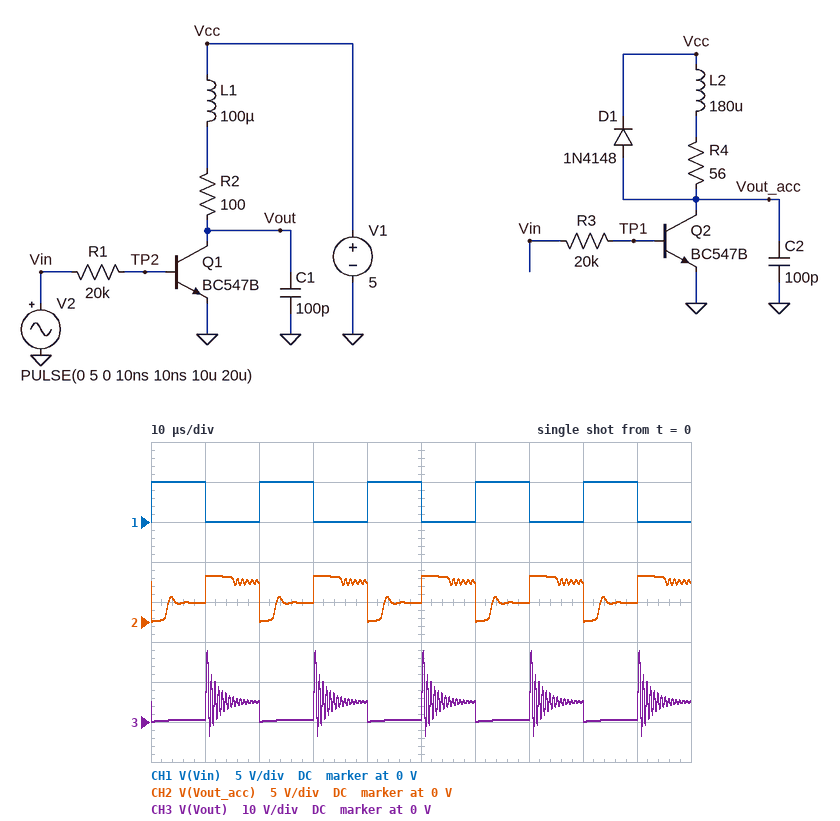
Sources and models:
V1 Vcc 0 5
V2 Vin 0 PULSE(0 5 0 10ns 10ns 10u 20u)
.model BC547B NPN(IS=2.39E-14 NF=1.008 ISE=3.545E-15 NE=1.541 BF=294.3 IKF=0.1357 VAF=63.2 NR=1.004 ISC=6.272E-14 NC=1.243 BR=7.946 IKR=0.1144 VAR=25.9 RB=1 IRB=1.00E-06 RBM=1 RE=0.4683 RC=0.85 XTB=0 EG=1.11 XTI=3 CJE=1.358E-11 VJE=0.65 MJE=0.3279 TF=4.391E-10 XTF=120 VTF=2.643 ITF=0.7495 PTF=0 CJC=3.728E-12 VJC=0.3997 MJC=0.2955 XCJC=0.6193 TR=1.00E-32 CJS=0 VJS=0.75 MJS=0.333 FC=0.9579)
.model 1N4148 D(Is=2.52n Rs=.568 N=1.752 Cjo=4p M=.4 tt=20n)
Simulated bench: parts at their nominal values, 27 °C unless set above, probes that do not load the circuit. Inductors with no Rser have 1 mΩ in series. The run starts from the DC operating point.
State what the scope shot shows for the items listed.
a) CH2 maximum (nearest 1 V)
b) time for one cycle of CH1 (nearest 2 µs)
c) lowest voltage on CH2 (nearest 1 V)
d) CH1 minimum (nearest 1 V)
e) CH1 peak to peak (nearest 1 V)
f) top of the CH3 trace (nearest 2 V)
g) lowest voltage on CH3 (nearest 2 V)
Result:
6 V
20 µs
0 V
0 V
5 V
18 V
-4 V
